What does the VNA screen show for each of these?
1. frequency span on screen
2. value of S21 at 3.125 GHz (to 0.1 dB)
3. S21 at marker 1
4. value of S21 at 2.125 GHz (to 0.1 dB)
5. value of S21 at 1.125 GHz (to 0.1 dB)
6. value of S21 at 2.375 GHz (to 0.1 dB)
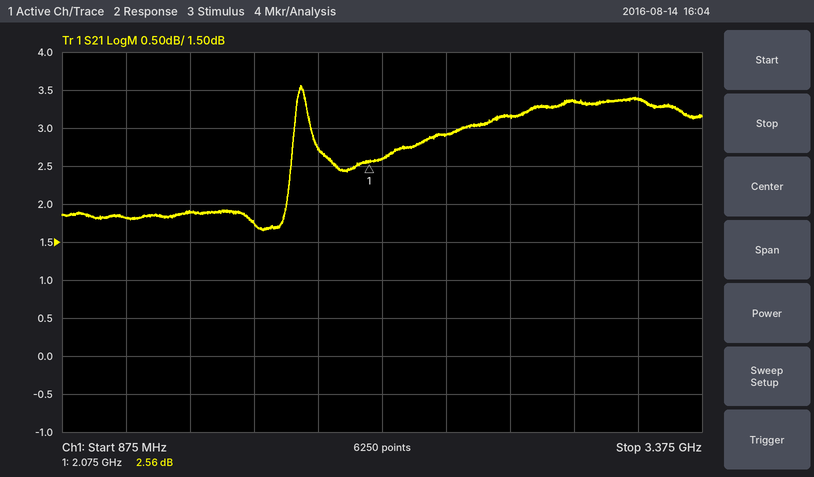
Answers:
2.5 GHz
3.4 dB
2.56 dB
2.6 dB
1.8 dB
2.9 dB
